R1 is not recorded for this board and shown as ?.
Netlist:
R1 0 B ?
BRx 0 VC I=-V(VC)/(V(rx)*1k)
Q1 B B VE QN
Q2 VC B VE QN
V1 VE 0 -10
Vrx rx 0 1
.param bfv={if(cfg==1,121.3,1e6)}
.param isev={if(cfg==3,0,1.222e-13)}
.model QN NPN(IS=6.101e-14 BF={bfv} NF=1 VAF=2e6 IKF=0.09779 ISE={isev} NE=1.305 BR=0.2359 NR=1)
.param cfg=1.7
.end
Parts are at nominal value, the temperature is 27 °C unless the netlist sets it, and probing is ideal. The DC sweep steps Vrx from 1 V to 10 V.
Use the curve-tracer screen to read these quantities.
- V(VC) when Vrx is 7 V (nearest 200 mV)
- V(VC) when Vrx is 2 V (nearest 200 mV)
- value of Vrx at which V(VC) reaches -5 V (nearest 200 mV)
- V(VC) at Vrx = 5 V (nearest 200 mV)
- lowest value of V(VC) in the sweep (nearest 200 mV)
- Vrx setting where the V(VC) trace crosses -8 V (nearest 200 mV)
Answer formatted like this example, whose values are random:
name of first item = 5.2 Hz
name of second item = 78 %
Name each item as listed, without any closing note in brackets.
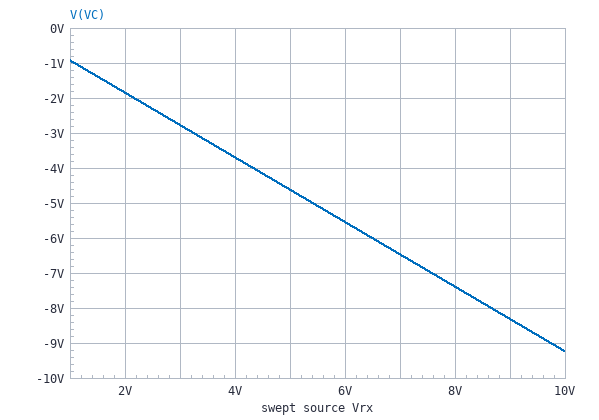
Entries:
V(VC) when Vrx is 7 V = -6.4 V
V(VC) when Vrx is 2 V = -1.8 V
value of Vrx at which V(VC) reaches -5 V = 5.4 V
V(VC) at Vrx = 5 V = -4.6 V
lowest value of V(VC) in the sweep = -9.2 V
Vrx setting where the V(VC) trace crosses -8 V = 8.6 V
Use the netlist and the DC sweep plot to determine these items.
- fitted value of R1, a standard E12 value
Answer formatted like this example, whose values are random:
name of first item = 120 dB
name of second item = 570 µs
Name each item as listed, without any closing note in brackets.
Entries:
fitted value of R1, a standard E12 value = 10 kΩ
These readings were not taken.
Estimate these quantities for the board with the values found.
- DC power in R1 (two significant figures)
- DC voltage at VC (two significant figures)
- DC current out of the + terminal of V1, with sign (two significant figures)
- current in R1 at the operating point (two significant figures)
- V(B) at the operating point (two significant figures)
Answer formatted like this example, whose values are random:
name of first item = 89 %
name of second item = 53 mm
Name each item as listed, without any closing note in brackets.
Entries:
DC power in R1 = 8.8 mW
DC voltage at VC = -920 mV
DC current out of the + terminal of V1, with sign = -1.9 mA
current in R1 at the operating point = 940 µA
V(B) at the operating point = -9.4 V
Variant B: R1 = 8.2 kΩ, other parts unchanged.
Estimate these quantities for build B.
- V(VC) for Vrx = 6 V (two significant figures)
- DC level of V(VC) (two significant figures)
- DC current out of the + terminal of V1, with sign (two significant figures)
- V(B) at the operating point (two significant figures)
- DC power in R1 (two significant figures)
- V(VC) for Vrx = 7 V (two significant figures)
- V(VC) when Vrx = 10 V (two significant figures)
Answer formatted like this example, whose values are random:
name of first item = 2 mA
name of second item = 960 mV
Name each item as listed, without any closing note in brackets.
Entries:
V(VC) for Vrx = 6 V = -6.8 V
DC level of V(VC) = -1.1 V
DC current out of the + terminal of V1, with sign = -2.3 mA
V(B) at the operating point = -9.4 V
DC power in R1 = 11 mW
V(VC) for Vrx = 7 V = -7.9 V
V(VC) when Vrx = 10 V = -9.9 V
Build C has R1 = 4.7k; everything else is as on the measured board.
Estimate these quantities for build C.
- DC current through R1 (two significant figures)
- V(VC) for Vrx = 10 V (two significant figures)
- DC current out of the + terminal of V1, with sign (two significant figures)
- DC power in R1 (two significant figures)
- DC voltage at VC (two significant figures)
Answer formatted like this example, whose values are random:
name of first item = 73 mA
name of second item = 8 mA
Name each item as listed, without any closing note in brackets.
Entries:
DC current through R1 = 2.0 mA
V(VC) for Vrx = 10 V = -9.9 V
DC current out of the + terminal of V1, with sign = -4.0 mA
DC power in R1 = 19 mW
DC voltage at VC = -2.0 V
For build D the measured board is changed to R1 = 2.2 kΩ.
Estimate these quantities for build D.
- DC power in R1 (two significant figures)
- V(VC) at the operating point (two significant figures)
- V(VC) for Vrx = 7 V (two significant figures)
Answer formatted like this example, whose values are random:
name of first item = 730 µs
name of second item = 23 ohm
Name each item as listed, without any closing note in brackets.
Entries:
DC power in R1 = 40 mW
V(VC) at the operating point = -4.2 V
V(VC) for Vrx = 7 V = -9.9 V
